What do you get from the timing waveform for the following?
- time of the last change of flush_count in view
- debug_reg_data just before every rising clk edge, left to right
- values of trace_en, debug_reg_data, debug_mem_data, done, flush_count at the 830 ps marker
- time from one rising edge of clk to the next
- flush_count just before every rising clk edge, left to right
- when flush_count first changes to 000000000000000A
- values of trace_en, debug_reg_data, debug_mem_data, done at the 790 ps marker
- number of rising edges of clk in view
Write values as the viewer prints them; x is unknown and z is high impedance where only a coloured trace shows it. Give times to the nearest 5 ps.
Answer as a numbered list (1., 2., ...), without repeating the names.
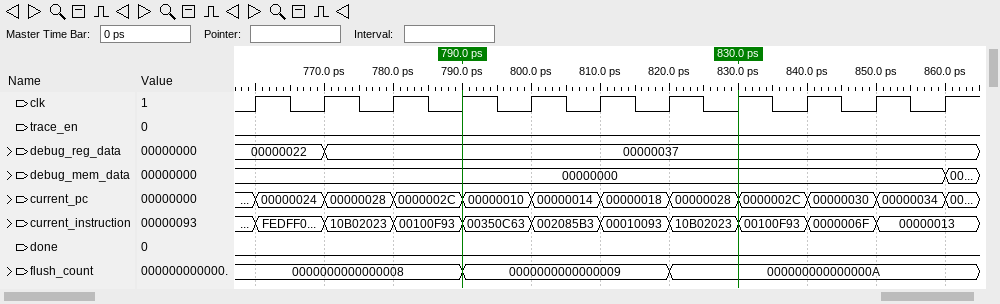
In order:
1. 820 ps
2. 00000022, 00000022, 00000037, 00000037, 00000037, 00000037, 00000037, 00000037, 00000037, 00000037, 00000037
3. trace_en=0, debug_reg_data=00000037, debug_mem_data=00000000, done=0, flush_count=000000000000000A
4. 10 ps
5. 0000000000000008, 0000000000000008, 0000000000000008, 0000000000000008, 0000000000000009, 0000000000000009, 0000000000000009, 000000000000000A, 000000000000000A, 000000000000000A, 000000000000000A
6. 820 ps
7. trace_en=0, debug_reg_data=00000037, debug_mem_data=00000000, done=0
8. 11
